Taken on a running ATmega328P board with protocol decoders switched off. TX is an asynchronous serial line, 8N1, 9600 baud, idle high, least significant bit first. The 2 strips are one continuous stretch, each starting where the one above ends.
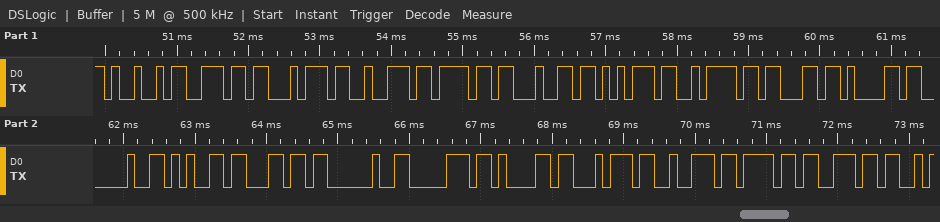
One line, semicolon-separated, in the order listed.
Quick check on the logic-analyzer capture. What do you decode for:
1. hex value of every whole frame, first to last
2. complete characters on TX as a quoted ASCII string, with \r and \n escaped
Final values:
49 6E 74 72 6F 64 75 7A 63 61 20 65 6C 20 70 61 74 72 6F 6E; "Introduzca el patron"
